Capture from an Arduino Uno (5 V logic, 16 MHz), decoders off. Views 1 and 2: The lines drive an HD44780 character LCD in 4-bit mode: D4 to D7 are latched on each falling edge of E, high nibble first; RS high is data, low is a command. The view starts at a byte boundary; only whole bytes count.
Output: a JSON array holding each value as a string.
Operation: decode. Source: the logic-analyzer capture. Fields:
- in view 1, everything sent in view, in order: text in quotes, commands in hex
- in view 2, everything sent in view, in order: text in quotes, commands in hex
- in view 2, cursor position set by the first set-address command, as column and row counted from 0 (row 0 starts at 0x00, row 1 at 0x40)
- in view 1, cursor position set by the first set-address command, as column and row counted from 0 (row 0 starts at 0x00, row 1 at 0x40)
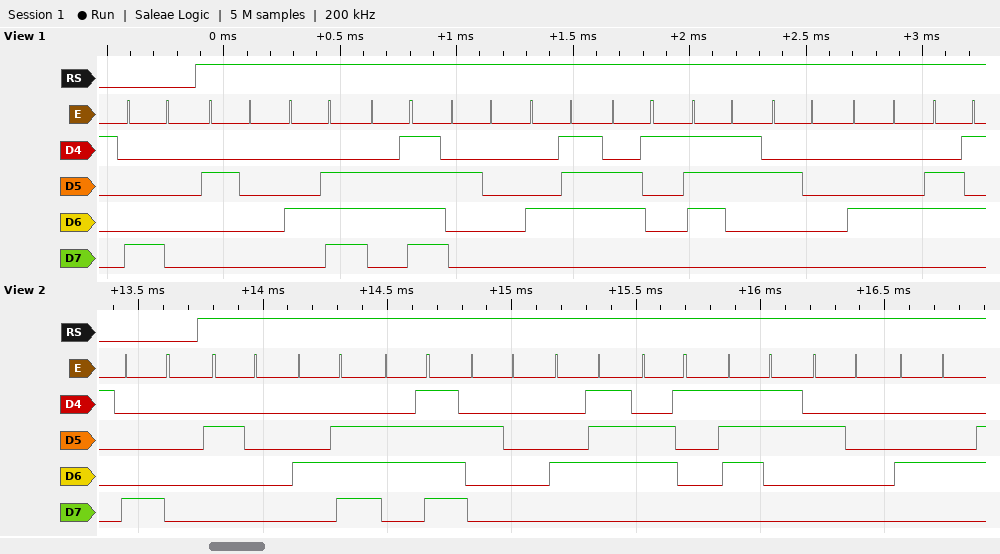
["0x80 \" No Gas De\"", "0x80 \" No Gas D\"", "column 0, row 0", "column 0, row 0"]
